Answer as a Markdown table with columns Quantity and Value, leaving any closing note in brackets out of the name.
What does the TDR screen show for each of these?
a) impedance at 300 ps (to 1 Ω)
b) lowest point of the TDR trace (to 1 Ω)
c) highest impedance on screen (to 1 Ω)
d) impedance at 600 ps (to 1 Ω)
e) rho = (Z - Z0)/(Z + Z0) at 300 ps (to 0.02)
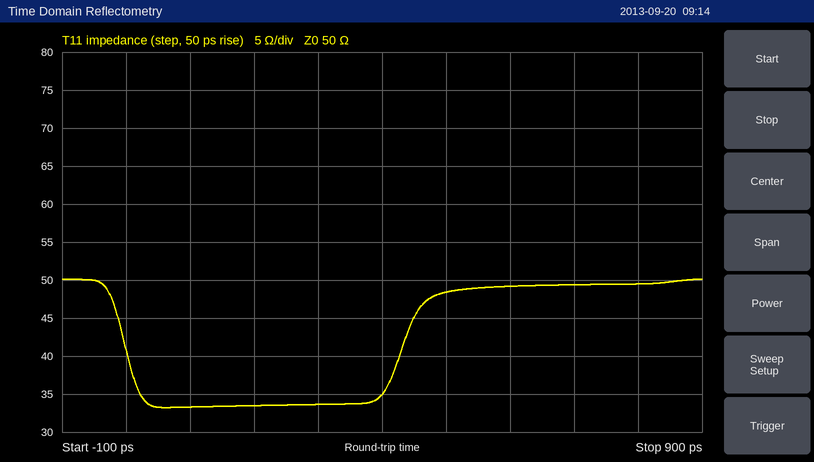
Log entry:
| Quantity | Value |
|---|---|
| impedance at 300 ps | 34 Ω |
| lowest point of the TDR trace | 33 Ω |
| highest impedance on screen | 50 Ω |
| impedance at 600 ps | 49 Ω |
| rho = (Z - Z0)/(Z + Z0) at 300 ps | -0.20 |
